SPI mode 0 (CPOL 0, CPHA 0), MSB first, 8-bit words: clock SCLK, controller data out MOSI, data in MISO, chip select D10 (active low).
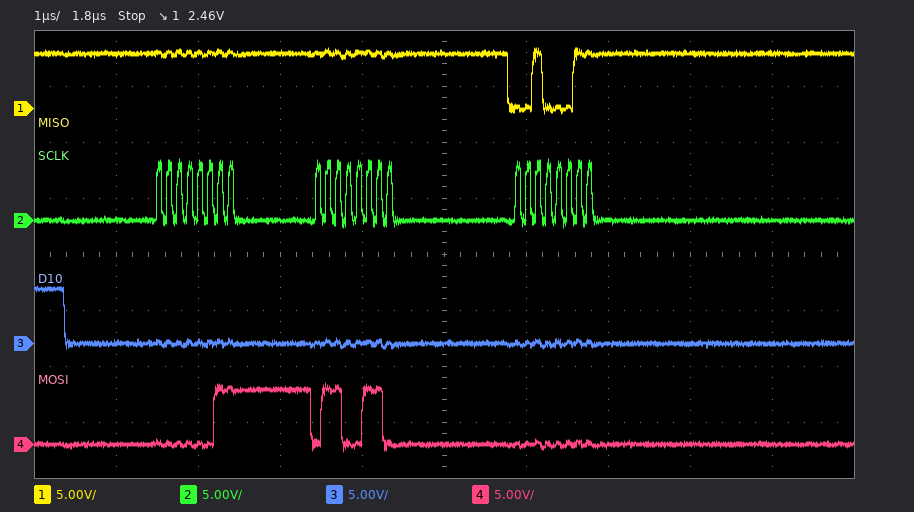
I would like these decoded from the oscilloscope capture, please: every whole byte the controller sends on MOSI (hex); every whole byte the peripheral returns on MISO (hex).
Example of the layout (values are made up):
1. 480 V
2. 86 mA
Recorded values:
1. 03 66 00
2. FF FF 23
